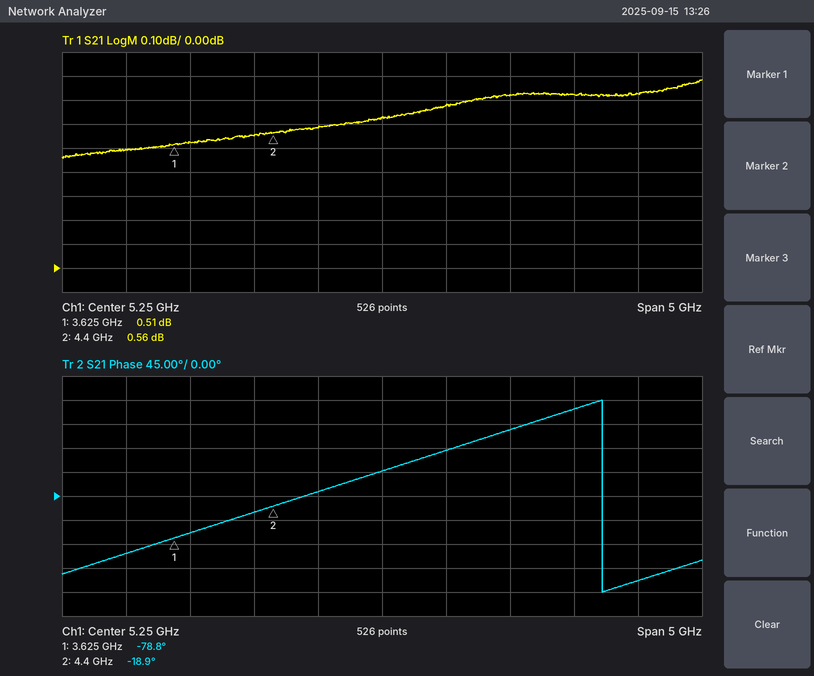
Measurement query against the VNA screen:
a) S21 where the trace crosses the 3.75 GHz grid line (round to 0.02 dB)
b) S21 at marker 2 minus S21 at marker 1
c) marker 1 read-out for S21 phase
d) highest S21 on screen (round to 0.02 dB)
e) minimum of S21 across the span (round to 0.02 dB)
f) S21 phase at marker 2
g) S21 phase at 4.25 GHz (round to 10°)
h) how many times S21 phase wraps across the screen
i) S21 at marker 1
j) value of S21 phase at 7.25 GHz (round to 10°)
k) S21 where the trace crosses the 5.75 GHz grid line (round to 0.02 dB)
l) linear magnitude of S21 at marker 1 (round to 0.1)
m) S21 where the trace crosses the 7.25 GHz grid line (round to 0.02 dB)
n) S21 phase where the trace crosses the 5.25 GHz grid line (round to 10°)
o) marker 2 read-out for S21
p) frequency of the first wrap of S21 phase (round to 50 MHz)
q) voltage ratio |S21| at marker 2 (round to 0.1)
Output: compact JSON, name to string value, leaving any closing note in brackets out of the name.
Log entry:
{"S21 where the trace crosses the 3.75 GHz grid line": "0.52 dB", "S21 at marker 2 minus S21 at marker 1": "0.05 dB", "marker 1 read-out for S21 phase": "-78.8°", "highest S21 on screen": "0.78 dB", "minimum of S21 across the span": "0.46 dB", "S21 phase at marker 2": "-18.9°", "S21 phase at 4.25 GHz": "-30°", "how many times S21 phase wraps across the screen": "1", "S21 at marker 1": "0.51 dB", "value of S21 phase at 7.25 GHz": "-160°", "S21 where the trace crosses the 5.75 GHz grid line": "0.68 dB", "linear magnitude of S21 at marker 1": "1.1", "S21 where the trace crosses the 7.25 GHz grid line": "0.72 dB", "S21 phase where the trace crosses the 5.25 GHz grid line": "50°", "marker 2 read-out for S21": "0.56 dB", "frequency of the first wrap of S21 phase": "6.95 GHz", "voltage ratio |S21| at marker 2": "1.1"}
